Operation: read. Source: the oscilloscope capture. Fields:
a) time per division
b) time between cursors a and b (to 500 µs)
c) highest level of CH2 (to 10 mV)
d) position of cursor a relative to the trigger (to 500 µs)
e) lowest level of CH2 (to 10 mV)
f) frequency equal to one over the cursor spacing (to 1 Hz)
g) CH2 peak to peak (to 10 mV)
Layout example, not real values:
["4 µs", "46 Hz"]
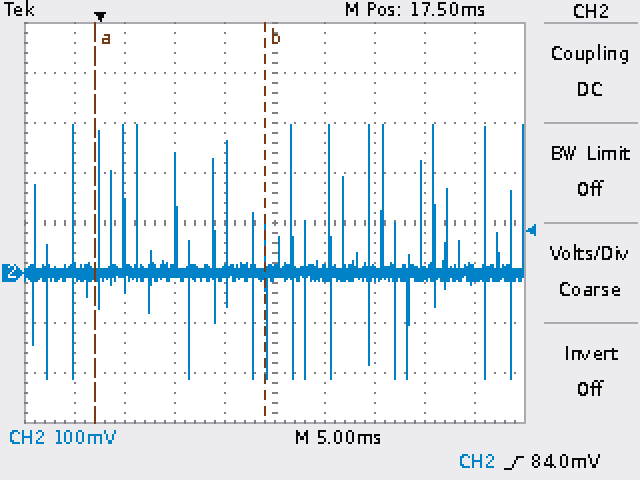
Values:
["5 ms", "17.0 ms", "300 mV", "-500 µs", "-210 mV", "59 Hz", "510 mV"]
